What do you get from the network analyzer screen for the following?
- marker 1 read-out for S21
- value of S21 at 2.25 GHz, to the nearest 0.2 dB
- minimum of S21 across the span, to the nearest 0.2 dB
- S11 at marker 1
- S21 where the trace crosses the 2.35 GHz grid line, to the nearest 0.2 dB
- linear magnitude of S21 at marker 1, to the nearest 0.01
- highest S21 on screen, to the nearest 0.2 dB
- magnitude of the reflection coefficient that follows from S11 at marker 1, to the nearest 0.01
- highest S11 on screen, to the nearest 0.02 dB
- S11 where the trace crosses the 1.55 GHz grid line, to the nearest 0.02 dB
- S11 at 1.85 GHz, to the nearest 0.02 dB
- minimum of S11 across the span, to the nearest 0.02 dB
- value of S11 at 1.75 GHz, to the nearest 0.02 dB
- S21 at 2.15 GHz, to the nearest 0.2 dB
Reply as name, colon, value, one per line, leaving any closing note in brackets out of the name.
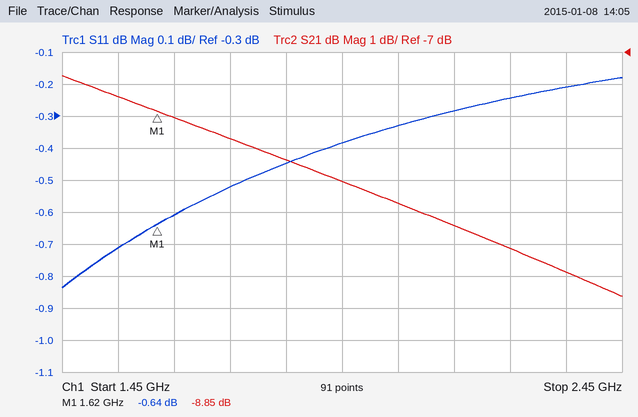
marker 1 read-out for S21: -8.85 dB
value of S21 at 2.25 GHz, to the nearest 0.2 dB: -13.2 dB
minimum of S21 across the span, to the nearest 0.2 dB: -14.6 dB
S11 at marker 1: -0.64 dB
S21 where the trace crosses the 2.35 GHz grid line, to the nearest 0.2 dB: -13.8 dB
linear magnitude of S21 at marker 1, to the nearest 0.01: 0.36
highest S21 on screen, to the nearest 0.2 dB: -7.8 dB
magnitude of the reflection coefficient that follows from S11 at marker 1, to the nearest 0.01: 0.93
highest S11 on screen, to the nearest 0.02 dB: -0.18 dB
S11 where the trace crosses the 1.55 GHz grid line, to the nearest 0.02 dB: -0.72 dB
S11 at 1.85 GHz, to the nearest 0.02 dB: -0.44 dB
minimum of S11 across the span, to the nearest 0.02 dB: -0.84 dB
value of S11 at 1.75 GHz, to the nearest 0.02 dB: -0.52 dB
S21 at 2.15 GHz, to the nearest 0.2 dB: -12.4 dB
